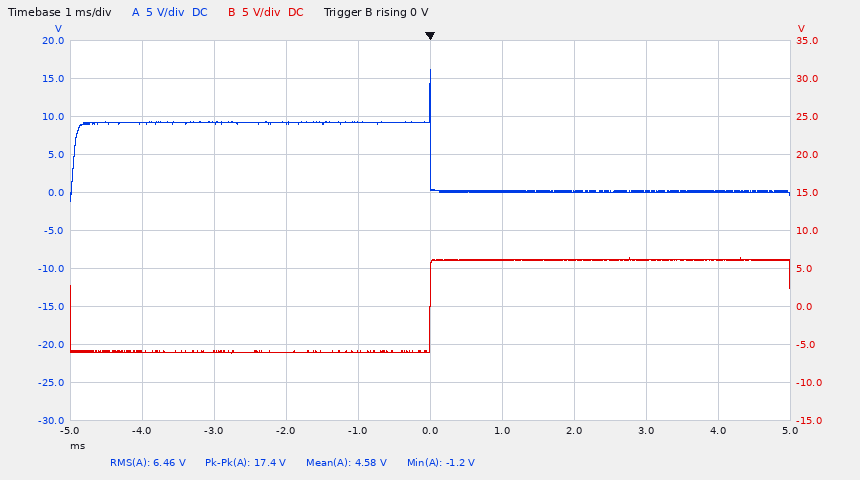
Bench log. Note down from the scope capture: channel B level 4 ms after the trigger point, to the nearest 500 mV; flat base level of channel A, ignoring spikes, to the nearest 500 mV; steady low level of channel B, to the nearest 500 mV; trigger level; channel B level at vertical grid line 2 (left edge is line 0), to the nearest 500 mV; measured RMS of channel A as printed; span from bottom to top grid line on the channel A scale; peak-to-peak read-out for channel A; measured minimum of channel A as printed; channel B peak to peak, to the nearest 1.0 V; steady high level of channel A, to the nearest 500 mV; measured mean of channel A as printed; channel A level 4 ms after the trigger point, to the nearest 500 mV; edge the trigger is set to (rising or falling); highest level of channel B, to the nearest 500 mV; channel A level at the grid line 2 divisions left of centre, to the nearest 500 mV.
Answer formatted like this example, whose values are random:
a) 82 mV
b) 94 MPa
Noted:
a) 6.0 V
b) 0.0 V
c) -6.0 V
d) 0 V
e) -6.0 V
f) 6.46 V
g) 50 V
h) 17.4 V
i) -1.2 V
j) 13.0 V
k) 9.0 V
l) 4.58 V
m) 0.0 V
n) rising
o) 6.5 V
p) 9.0 V
